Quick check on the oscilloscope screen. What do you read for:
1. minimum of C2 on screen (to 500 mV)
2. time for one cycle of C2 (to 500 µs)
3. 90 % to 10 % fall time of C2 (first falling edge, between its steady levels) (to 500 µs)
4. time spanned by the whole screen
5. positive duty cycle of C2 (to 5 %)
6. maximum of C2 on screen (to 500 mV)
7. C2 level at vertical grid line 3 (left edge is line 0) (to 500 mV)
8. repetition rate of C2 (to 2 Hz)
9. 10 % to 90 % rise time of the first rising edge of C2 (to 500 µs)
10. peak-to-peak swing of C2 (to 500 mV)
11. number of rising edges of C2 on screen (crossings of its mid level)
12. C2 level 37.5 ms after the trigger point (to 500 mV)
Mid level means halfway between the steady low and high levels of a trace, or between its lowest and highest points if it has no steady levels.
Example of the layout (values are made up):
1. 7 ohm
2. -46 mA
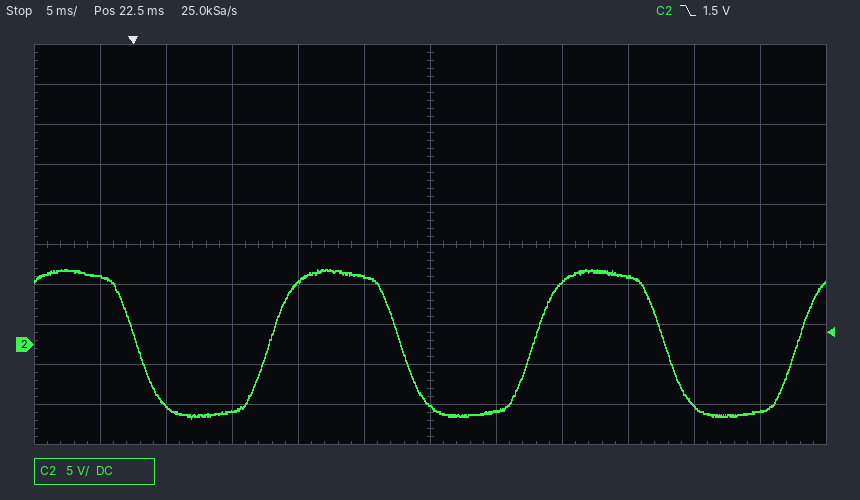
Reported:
1. -9.0 V
2. 20.0 ms
3. 3.5 ms
4. 60 ms
5. 50 %
6. 9.5 V
7. -8.5 V
8. 50 Hz
9. 3.5 ms
10. 18.5 V
11. 3
12. 8.5 V
